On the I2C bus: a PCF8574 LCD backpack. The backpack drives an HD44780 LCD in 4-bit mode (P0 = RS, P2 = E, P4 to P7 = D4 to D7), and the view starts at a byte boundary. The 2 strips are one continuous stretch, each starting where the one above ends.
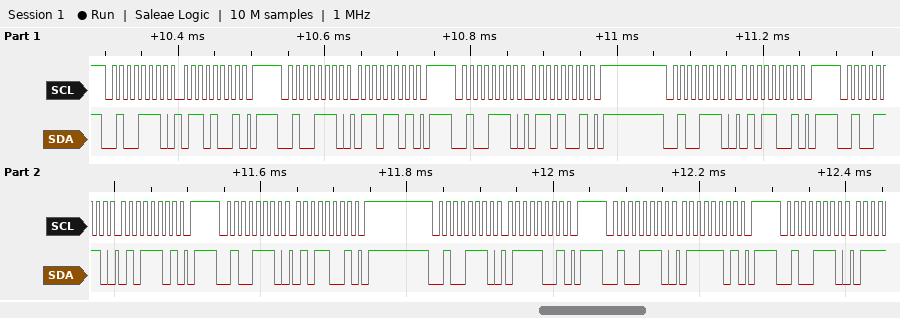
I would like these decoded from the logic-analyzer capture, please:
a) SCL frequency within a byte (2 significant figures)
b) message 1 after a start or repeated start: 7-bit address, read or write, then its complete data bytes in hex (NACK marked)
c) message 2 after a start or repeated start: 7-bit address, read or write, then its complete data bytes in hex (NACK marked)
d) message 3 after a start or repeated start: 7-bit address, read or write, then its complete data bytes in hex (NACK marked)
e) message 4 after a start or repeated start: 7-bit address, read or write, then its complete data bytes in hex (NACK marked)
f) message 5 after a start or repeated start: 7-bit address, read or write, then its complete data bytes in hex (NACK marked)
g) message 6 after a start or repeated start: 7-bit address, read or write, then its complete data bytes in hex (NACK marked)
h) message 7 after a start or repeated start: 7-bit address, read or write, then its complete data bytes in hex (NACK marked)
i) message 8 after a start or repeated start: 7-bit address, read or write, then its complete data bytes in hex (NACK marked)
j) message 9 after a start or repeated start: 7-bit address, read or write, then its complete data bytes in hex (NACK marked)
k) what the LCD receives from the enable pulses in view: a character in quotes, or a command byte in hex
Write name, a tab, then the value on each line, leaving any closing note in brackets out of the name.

SCL frequency within a byte	100 kHz
message 1 after a start or repeated start: 7-bit address, read or write, then its complete data bytes in hex	0x27 write: 69
message 2 after a start or repeated start: 7-bit address, read or write, then its complete data bytes in hex	0x27 write: 6D
message 3 after a start or repeated start: 7-bit address, read or write, then its complete data bytes in hex	0x27 write: 69
message 4 after a start or repeated start: 7-bit address, read or write, then its complete data bytes in hex	0x27 write: 59
message 5 after a start or repeated start: 7-bit address, read or write, then its complete data bytes in hex	0x27 write: 5D
message 6 after a start or repeated start: 7-bit address, read or write, then its complete data bytes in hex	0x27 write: 59
message 7 after a start or repeated start: 7-bit address, read or write, then its complete data bytes in hex	0x27 write: 79
message 8 after a start or repeated start: 7-bit address, read or write, then its complete data bytes in hex	0x27 write: 7D
message 9 after a start or repeated start: 7-bit address, read or write, then its complete data bytes in hex	0x27 write
what the LCD receives from the enable pulses in view: a character in quotes, or a command byte in hex	'e'
